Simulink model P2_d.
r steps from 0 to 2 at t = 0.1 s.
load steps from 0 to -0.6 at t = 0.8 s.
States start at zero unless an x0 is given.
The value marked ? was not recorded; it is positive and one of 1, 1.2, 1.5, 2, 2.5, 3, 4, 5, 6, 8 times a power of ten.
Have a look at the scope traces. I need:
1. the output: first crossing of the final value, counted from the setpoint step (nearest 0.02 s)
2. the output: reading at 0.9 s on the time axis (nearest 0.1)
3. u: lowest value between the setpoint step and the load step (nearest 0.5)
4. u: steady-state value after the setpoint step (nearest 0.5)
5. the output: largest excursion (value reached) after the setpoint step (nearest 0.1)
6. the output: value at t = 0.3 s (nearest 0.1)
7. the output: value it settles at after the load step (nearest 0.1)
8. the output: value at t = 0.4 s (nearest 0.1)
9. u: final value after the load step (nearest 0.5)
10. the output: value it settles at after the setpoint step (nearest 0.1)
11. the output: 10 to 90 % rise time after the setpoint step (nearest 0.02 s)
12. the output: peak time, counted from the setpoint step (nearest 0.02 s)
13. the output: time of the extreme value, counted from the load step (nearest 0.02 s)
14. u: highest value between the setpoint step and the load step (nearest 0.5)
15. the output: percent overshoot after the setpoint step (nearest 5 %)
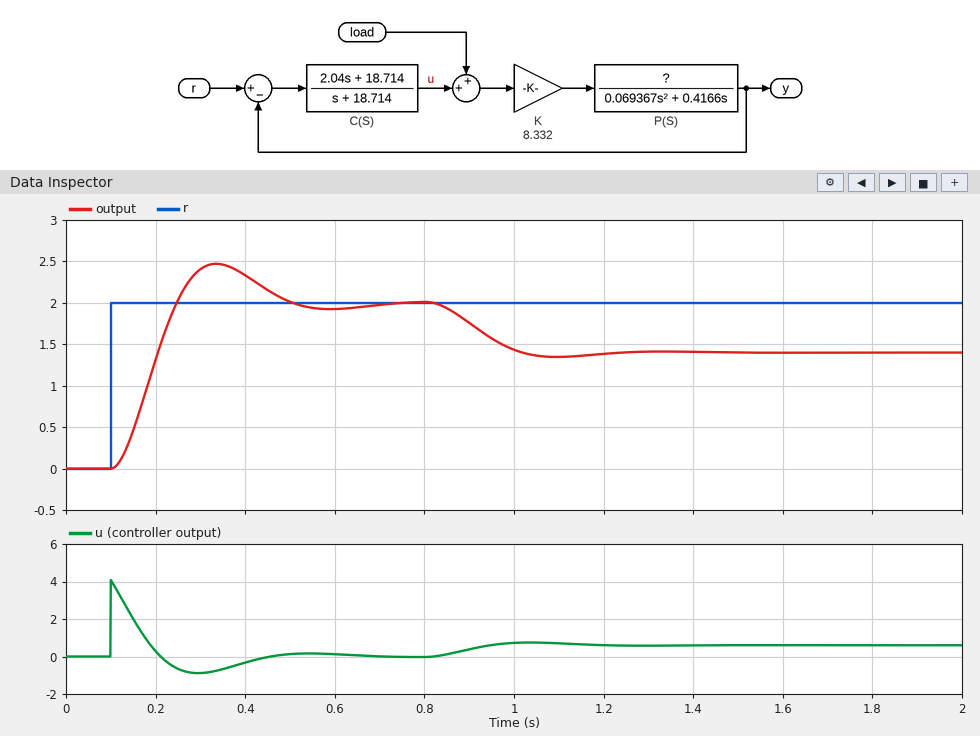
0.14 s
1.8
-1.0
0.0
2.5
2.4
1.4
2.3
0.5
2.0
0.10 s
0.24 s
0.30 s
4.0
25 %
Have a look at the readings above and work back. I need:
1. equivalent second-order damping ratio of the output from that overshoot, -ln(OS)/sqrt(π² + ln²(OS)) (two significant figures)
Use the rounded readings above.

0.40
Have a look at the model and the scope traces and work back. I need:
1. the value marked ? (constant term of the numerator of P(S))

1
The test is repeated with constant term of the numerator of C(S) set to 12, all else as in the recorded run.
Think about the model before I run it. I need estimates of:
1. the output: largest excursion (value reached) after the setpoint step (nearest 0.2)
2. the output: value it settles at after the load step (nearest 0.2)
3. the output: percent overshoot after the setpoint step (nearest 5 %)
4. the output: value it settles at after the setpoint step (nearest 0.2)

2.2
1.0
10 %
2.0
